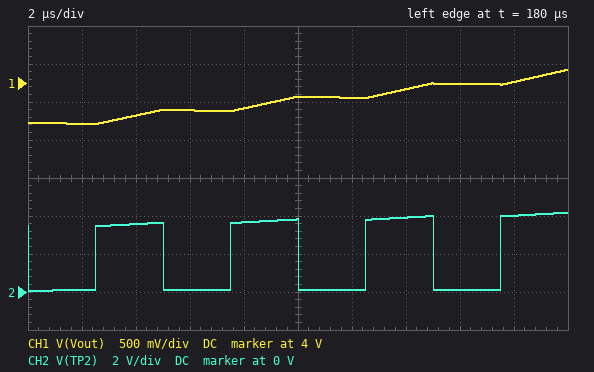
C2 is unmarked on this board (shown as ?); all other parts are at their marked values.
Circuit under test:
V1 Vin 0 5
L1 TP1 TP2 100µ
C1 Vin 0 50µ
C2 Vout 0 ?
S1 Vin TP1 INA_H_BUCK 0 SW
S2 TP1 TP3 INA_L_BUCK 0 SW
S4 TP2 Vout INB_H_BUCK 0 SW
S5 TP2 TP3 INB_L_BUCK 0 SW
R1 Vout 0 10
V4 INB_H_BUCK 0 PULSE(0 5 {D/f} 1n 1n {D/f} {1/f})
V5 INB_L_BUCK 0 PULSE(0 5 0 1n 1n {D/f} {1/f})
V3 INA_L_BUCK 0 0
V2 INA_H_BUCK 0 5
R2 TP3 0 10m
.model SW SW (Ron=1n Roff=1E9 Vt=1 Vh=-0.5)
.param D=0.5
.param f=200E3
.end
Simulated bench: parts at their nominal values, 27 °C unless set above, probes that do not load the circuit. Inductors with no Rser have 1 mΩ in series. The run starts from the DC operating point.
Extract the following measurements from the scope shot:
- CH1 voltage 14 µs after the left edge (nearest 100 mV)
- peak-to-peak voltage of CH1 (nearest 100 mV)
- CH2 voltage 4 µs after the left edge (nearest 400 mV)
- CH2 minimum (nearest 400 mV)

3.9 V
700 mV
3.6 V
0 V
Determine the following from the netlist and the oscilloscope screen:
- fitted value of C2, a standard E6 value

100 µF
